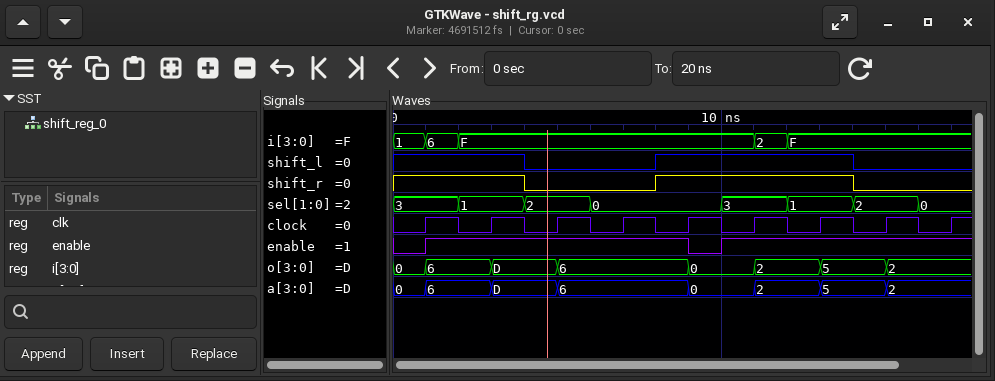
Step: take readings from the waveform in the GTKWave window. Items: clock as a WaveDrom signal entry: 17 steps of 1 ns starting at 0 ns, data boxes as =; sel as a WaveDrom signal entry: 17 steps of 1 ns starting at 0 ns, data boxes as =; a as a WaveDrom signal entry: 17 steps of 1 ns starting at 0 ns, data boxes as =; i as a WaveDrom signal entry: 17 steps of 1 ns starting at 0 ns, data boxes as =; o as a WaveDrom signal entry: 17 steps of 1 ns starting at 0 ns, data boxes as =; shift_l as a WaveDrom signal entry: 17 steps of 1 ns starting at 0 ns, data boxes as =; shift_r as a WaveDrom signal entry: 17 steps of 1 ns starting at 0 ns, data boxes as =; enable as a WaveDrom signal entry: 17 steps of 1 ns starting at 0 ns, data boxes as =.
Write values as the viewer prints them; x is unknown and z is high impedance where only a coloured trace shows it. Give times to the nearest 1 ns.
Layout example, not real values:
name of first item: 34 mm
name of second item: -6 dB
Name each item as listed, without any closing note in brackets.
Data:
clock as a WaveDrom signal entry: 17 steps of 1 ns starting at 0 ns, data boxes as =: {name: 'clock', wave: '01010101010101010'}
sel as a WaveDrom signal entry: 17 steps of 1 ns starting at 0 ns, data boxes as =: {name: 'sel', wave: '=.=.=.=...=.=.=.=', data: '3 1 2 0 3 1 2 0'}
a as a WaveDrom signal entry: 17 steps of 1 ns starting at 0 ns, data boxes as =: {name: 'a', wave: '==.=.=...=.=.=.=.', data: '0 6 D 6 0 2 5 2'}
i as a WaveDrom signal entry: 17 steps of 1 ns starting at 0 ns, data boxes as =: {name: 'i', wave: '===........==....', data: '1 6 F 2 F'}
o as a WaveDrom signal entry: 17 steps of 1 ns starting at 0 ns, data boxes as =: {name: 'o', wave: '==.=.=...=.=.=.=.', data: '0 6 D 6 0 2 5 2'}
shift_l as a WaveDrom signal entry: 17 steps of 1 ns starting at 0 ns, data boxes as =: {name: 'shift_l', wave: '1...0...1.....0..'}
shift_r as a WaveDrom signal entry: 17 steps of 1 ns starting at 0 ns, data boxes as =: {name: 'shift_r', wave: '1...0...1.....0..'}
enable as a WaveDrom signal entry: 17 steps of 1 ns starting at 0 ns, data boxes as =: {name: 'enable', wave: '01.......01......'}
